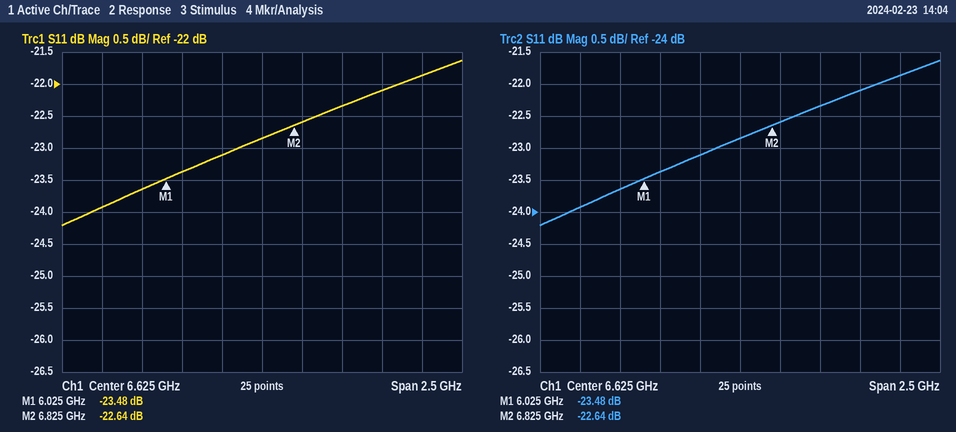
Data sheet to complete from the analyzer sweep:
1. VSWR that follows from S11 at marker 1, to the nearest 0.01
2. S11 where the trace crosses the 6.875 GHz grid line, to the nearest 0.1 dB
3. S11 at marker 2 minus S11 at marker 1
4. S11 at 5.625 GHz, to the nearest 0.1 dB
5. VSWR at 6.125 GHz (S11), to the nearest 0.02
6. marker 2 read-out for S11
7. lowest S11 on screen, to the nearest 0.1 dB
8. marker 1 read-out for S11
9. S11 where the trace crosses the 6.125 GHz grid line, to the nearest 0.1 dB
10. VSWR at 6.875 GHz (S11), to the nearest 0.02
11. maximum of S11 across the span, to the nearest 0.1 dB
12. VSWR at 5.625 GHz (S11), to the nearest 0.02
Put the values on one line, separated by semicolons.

1.14; -22.6 dB; 0.84 dB; -23.9 dB; 1.14; -22.64 dB; -24.2 dB; -23.48 dB; -23.4 dB; 1.16; -21.6 dB; 1.14
